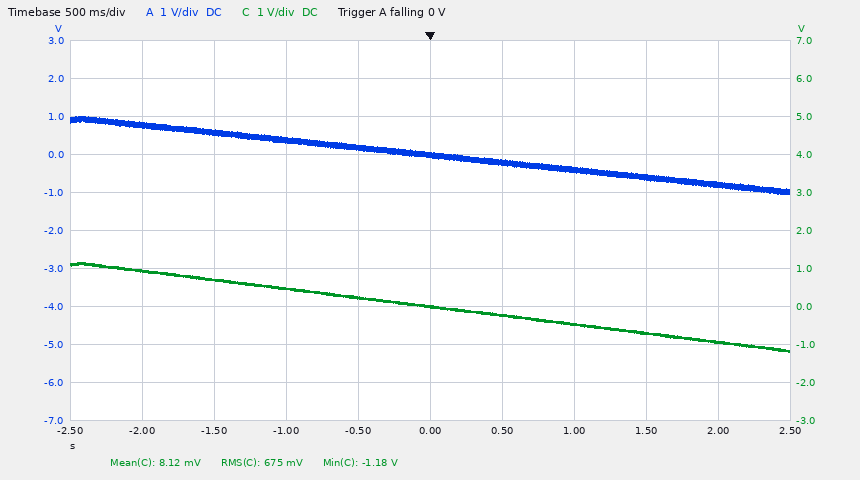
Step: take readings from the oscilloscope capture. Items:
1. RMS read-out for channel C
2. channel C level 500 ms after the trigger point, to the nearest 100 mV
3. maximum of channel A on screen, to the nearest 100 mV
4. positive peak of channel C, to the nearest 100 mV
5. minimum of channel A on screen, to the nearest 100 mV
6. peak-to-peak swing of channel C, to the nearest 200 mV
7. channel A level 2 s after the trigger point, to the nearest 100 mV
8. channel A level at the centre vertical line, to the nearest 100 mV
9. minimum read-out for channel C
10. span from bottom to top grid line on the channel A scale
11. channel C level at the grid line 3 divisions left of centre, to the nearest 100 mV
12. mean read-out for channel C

675 mV
-200 mV
1.0 V
1.2 V
-1.0 V
2.4 V
-800 mV
0.0 V
-1.18 V
10 V
700 mV
8.12 mV
